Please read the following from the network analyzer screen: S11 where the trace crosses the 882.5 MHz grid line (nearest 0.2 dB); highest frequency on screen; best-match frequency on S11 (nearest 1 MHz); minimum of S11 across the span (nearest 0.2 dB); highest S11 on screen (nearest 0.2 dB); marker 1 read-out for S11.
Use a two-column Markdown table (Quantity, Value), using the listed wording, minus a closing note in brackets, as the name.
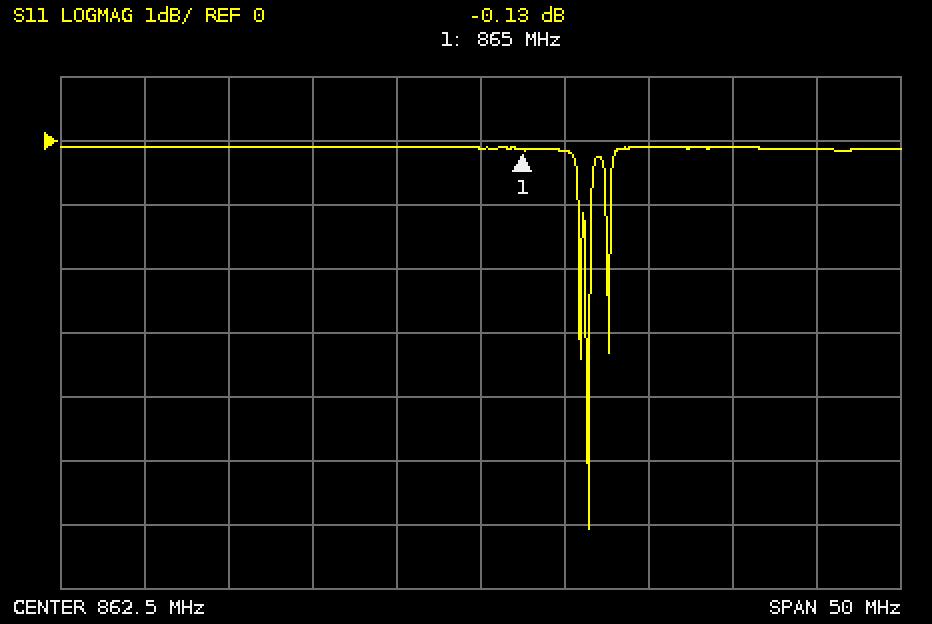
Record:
| Quantity | Value |
|---|---|
| S11 where the trace crosses the 882.5 MHz grid line | -0.2 dB |
| highest frequency on screen | 887.5 MHz |
| best-match frequency on S11 | 869 MHz |
| minimum of S11 across the span | -6.0 dB |
| highest S11 on screen | 0.0 dB |
| marker 1 read-out for S11 | -0.13 dB |
